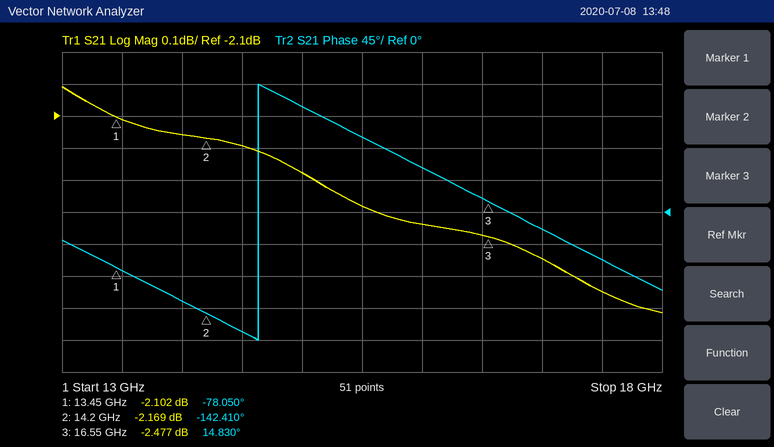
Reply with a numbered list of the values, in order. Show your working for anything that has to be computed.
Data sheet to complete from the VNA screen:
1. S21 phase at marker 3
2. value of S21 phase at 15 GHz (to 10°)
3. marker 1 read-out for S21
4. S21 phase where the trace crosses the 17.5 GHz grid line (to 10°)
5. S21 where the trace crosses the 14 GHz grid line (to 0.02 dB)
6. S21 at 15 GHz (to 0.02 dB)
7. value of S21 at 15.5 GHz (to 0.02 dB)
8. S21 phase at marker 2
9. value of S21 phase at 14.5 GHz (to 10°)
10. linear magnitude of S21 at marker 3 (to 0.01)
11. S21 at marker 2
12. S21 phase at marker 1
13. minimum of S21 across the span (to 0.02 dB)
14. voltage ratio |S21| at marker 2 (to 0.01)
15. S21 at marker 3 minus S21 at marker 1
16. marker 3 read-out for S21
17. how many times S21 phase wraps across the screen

1. 14.830°
2. 150°
3. -2.102 dB
4. -70°
5. -2.16 dB
6. -2.28 dB
7. -2.38 dB
8. -142.410°
9. -170°
10. 10^(-2.477/20) ≈ 0.75
11. -2.169 dB
12. -78.050°
13. -2.72 dB
14. 10^(-2.169/20) ≈ 0.78
15. -2.477 − (-2.102) = -0.375 dB
16. -2.477 dB
17. 1
